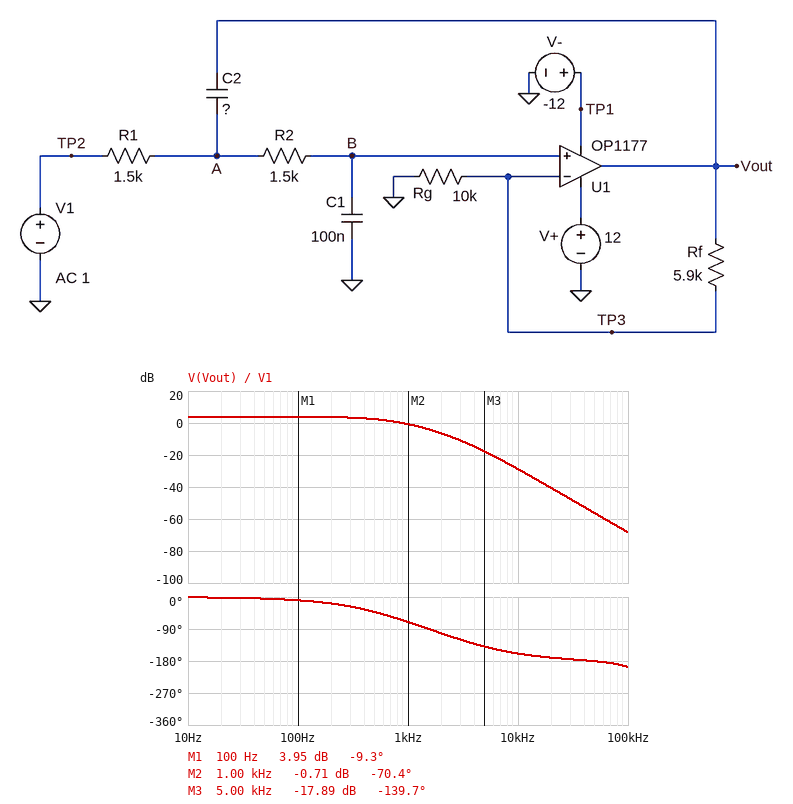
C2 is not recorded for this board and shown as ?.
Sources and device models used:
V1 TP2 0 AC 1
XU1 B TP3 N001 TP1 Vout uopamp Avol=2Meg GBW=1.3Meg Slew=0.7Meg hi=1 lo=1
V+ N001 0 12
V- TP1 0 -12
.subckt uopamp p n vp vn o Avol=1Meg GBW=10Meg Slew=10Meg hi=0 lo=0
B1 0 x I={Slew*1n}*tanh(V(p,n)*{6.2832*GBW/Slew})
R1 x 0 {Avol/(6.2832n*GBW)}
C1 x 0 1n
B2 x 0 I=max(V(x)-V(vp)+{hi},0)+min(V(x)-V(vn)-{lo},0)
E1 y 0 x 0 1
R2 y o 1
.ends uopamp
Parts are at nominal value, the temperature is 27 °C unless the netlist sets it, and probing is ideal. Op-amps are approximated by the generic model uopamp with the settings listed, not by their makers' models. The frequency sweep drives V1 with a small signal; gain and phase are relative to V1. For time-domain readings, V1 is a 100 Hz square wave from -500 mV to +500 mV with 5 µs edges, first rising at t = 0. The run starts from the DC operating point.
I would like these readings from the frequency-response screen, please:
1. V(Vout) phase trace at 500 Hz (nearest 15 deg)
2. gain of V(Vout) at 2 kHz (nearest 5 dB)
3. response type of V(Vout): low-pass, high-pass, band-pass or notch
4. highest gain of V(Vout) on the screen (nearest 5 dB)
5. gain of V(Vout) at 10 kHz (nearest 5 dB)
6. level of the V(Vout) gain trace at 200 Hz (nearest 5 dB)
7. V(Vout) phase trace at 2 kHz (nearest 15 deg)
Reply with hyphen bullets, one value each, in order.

- -45 deg
- -5 dB
- low-pass
- 5 dB
- -30 dB
- 5 dB
- -105 deg
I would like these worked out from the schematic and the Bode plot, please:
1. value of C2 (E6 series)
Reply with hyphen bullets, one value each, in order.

- 47 nF
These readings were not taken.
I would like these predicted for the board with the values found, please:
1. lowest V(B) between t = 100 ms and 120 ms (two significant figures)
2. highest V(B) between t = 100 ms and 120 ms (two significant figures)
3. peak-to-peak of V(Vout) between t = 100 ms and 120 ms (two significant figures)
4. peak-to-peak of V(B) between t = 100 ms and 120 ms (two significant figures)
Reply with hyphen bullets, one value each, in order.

- -500 mV
- 500 mV
- 1.6 V
- 1.0 V
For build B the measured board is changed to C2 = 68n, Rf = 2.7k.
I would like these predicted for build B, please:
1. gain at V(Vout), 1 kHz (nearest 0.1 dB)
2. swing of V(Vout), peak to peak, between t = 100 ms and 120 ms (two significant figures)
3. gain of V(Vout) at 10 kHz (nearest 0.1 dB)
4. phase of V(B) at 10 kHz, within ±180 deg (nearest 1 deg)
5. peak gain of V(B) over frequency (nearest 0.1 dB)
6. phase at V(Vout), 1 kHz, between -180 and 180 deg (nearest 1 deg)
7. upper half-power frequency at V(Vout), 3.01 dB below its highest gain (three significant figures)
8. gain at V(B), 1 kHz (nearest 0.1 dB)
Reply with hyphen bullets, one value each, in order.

- -2.8 dB
- 1.3 V
- -33.8 dB
- -164 deg
- 0 dB
- -77 deg
- 723 Hz
- -4.9 dB
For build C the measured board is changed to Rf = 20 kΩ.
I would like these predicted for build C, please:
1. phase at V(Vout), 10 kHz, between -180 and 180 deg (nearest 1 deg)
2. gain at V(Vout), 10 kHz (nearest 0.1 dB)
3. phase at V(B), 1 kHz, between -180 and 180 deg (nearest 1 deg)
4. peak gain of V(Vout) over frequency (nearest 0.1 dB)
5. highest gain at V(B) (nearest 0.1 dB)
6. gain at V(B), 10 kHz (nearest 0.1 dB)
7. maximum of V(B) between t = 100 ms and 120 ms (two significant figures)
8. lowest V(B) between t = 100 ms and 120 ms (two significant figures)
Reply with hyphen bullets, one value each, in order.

- -168 deg
- -23.0 dB
- -60 deg
- 9.5 dB
- 0 dB
- -32.5 dB
- 520 mV
- -520 mV
